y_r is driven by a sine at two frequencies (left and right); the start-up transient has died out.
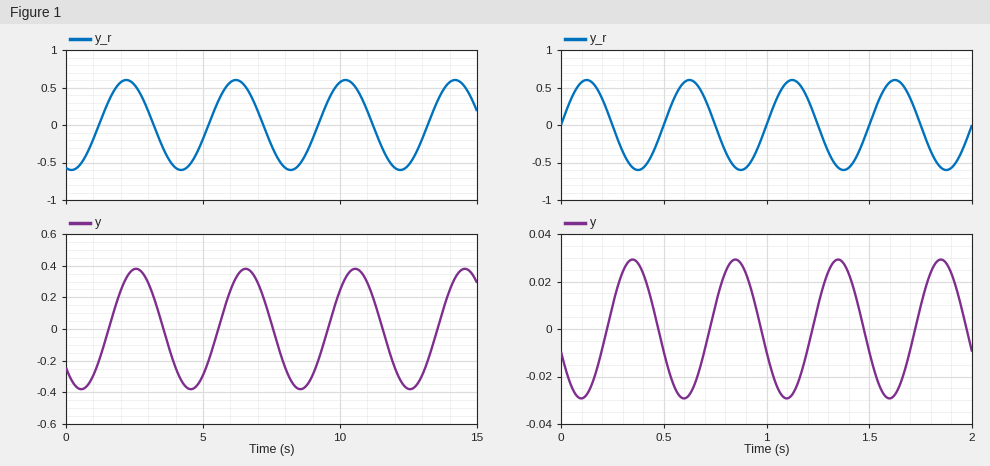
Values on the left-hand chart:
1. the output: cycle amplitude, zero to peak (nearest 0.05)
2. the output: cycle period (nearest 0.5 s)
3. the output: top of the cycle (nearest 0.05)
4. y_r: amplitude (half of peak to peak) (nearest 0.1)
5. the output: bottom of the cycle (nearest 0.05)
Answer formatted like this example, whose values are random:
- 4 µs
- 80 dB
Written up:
- 0.40
- 4.0 s
- 0.40
- 0.6
- -0.40
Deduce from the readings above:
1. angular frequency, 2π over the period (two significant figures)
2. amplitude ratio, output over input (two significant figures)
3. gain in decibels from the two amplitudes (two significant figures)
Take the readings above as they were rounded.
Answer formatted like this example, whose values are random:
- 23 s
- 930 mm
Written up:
- 1.6 rad/s
- 0.67
- -3.5 dB
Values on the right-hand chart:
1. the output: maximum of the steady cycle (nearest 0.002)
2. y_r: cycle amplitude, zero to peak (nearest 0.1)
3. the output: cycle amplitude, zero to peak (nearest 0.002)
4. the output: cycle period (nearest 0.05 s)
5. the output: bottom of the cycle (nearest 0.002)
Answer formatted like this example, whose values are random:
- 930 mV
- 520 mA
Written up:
- 0.030
- 0.6
- 0.030
- 0.50 s
- -0.030
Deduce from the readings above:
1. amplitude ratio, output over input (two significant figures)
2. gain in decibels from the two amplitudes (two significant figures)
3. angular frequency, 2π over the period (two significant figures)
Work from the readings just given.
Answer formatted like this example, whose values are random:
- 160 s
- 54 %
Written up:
- 0.050
- -26 dB
- 13 rad/s
